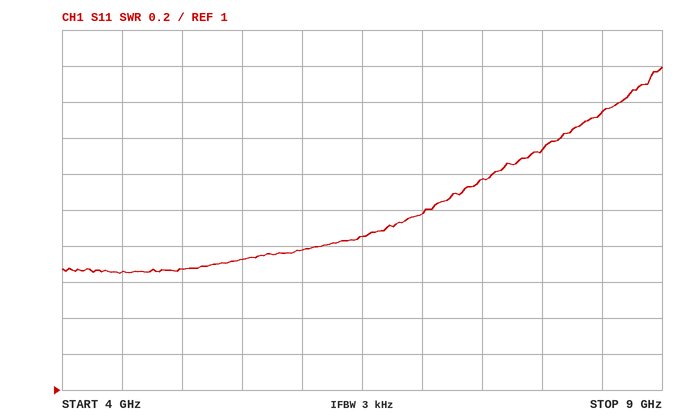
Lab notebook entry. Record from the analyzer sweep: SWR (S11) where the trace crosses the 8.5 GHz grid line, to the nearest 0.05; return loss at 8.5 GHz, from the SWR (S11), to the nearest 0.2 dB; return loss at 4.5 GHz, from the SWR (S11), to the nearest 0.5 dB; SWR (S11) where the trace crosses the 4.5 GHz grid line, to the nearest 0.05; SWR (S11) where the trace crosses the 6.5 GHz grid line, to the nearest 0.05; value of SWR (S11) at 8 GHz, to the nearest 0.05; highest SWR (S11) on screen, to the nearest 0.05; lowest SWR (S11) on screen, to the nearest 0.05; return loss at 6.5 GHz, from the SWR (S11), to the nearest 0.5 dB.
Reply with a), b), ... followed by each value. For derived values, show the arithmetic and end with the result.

a) 2.55
b) −20 log10((2.55 − 1)/(2.55 + 1)) ≈ 7.2 dB
c) −20 log10((1.65 − 1)/(1.65 + 1)) ≈ 12.2 dB, so 12.0 dB to the nearest 0.5 dB
d) 1.65
e) 1.85
f) 2.35
g) 2.80
h) 1.65
i) −20 log10((1.85 − 1)/(1.85 + 1)) ≈ 10.5 dB
